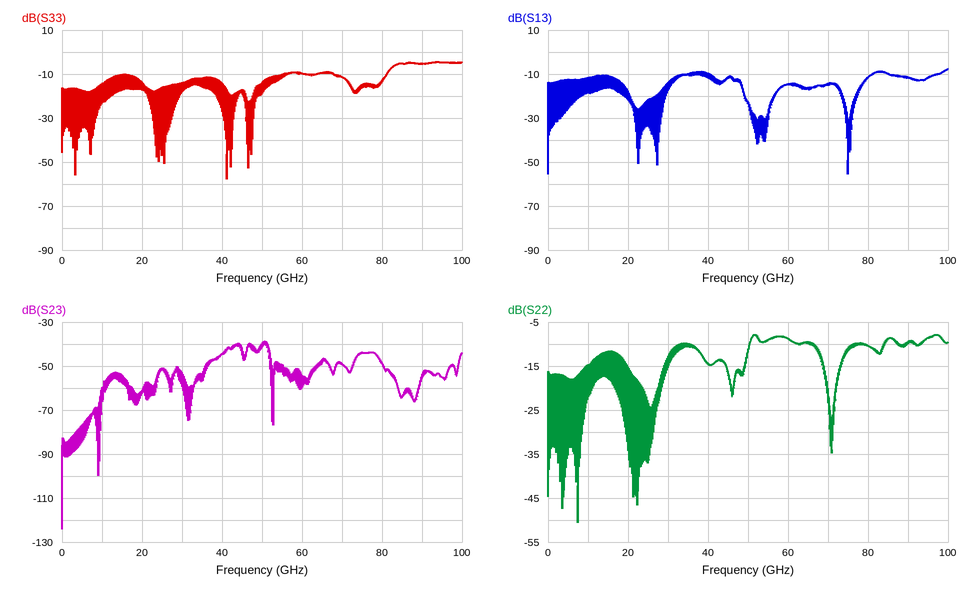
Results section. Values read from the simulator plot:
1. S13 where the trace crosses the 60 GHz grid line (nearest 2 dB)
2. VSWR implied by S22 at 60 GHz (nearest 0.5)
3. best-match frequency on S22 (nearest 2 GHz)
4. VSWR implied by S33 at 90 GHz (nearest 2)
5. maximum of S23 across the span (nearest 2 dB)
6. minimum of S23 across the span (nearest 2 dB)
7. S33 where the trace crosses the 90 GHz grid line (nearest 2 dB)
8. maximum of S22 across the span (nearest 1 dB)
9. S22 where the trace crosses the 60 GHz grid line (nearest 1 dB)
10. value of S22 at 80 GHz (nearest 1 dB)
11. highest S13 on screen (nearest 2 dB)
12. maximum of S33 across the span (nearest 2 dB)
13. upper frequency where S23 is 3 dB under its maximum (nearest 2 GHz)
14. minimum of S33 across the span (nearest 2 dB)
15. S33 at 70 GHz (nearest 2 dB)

-14 dB
2.0
8 GHz
4
-38 dB
-124 dB
-6 dB
-8 dB
-9 dB
-10 dB
-8 dB
-4 dB
52 GHz
-58 dB
-12 dB
